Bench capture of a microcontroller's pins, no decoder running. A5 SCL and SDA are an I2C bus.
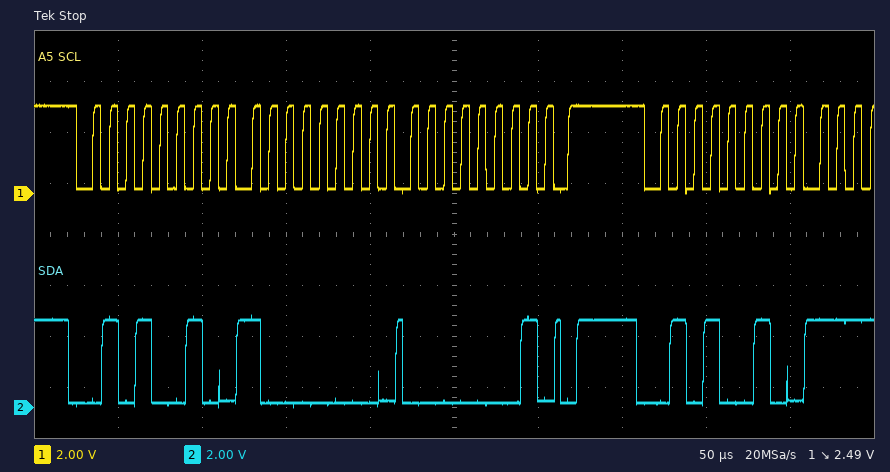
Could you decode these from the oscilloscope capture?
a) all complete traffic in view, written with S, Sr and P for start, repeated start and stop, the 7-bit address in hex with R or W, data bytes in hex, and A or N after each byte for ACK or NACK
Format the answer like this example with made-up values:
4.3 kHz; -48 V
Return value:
S 29W A 80 A 01 A P S 29W A
